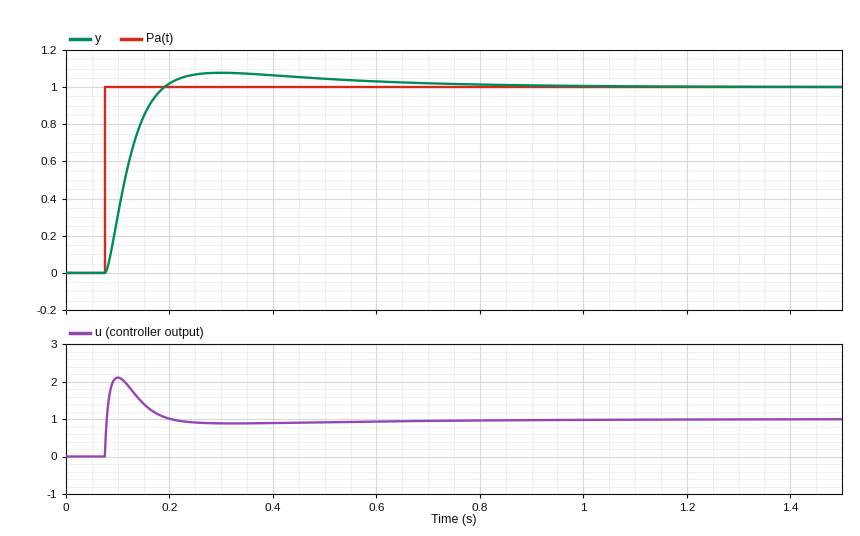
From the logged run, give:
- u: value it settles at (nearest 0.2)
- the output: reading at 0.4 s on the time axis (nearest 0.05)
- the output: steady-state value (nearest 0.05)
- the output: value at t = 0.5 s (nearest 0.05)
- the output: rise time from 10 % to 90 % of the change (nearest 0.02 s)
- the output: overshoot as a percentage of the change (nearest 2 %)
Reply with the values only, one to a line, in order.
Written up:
1.0
1.05
1.00
1.05
0.08 s
8 %
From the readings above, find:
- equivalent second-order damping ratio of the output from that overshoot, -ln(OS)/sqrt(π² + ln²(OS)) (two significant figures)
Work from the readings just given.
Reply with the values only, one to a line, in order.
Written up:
0.63
